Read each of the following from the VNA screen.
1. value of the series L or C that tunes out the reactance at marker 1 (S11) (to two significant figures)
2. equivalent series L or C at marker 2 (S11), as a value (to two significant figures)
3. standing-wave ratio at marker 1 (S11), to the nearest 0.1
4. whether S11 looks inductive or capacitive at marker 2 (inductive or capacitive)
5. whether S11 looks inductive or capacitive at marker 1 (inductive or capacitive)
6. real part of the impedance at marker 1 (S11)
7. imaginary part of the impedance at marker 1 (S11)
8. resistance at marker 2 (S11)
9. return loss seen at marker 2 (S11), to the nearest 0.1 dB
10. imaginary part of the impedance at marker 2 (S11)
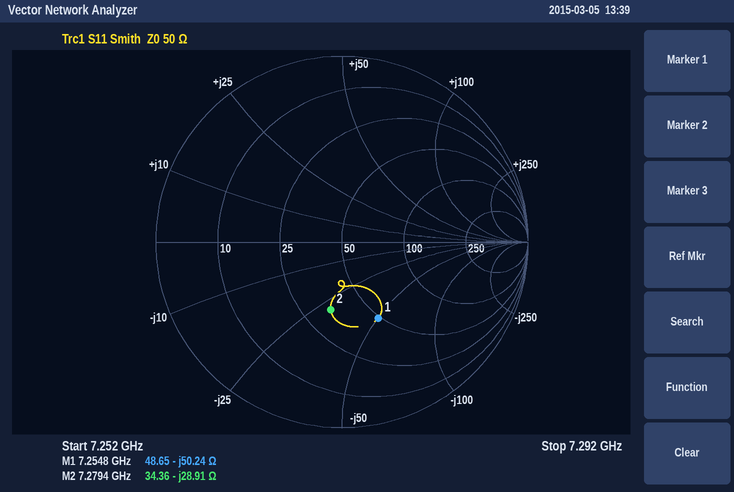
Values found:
1.1 nH
760 fF
2.7
capacitive
capacitive
48.65 Ω
-50.24 Ω
34.36 Ω
8.7 dB
-28.91 Ω
